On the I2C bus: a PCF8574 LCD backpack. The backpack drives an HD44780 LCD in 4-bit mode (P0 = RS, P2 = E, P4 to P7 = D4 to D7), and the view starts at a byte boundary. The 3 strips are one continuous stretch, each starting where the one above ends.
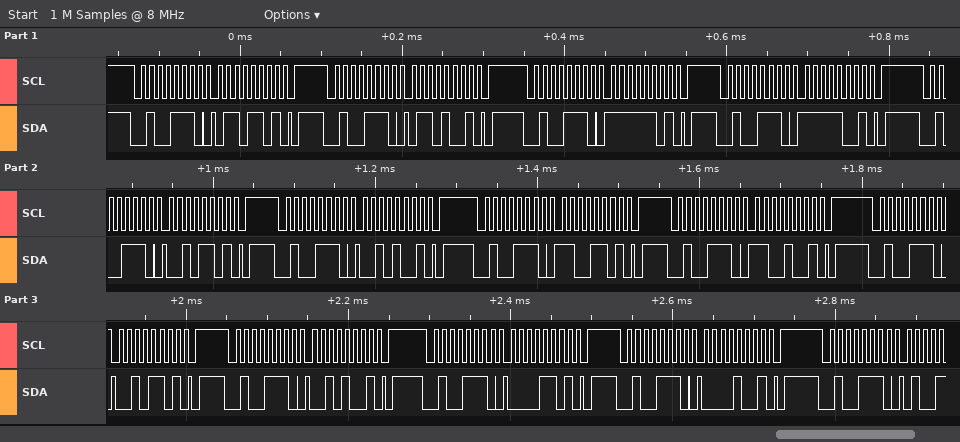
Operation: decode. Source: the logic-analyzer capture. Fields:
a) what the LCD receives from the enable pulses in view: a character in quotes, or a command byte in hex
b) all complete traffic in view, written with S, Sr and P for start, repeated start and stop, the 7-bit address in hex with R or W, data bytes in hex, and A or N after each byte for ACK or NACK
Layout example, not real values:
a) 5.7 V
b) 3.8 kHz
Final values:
a) 'o' ',' ' '
b) S 27W A 6D A P S 27W A 69 A P S 27W A FD A P S 27W A F9 A P S 27W A 2D A P S 27W A 29 A P S 27W A CD A P S 27W A C9 A P S 27W A 2D A P S 27W A 29 A P S 27W A 0D A P S 27W A 09 A P S 27W A
